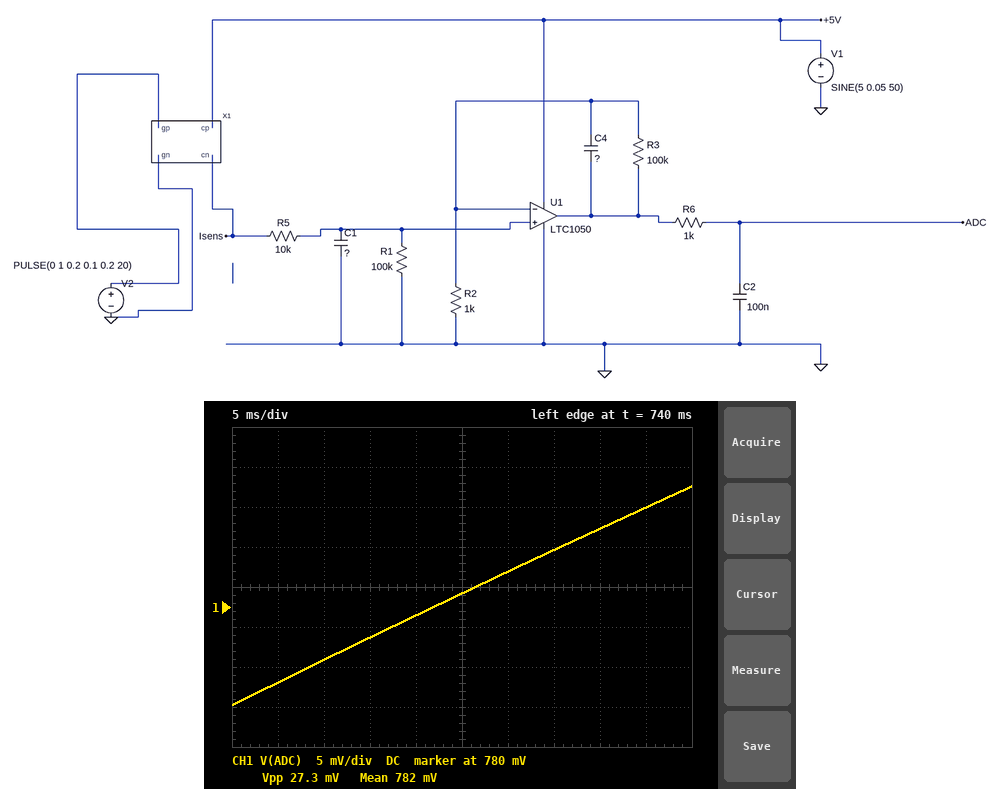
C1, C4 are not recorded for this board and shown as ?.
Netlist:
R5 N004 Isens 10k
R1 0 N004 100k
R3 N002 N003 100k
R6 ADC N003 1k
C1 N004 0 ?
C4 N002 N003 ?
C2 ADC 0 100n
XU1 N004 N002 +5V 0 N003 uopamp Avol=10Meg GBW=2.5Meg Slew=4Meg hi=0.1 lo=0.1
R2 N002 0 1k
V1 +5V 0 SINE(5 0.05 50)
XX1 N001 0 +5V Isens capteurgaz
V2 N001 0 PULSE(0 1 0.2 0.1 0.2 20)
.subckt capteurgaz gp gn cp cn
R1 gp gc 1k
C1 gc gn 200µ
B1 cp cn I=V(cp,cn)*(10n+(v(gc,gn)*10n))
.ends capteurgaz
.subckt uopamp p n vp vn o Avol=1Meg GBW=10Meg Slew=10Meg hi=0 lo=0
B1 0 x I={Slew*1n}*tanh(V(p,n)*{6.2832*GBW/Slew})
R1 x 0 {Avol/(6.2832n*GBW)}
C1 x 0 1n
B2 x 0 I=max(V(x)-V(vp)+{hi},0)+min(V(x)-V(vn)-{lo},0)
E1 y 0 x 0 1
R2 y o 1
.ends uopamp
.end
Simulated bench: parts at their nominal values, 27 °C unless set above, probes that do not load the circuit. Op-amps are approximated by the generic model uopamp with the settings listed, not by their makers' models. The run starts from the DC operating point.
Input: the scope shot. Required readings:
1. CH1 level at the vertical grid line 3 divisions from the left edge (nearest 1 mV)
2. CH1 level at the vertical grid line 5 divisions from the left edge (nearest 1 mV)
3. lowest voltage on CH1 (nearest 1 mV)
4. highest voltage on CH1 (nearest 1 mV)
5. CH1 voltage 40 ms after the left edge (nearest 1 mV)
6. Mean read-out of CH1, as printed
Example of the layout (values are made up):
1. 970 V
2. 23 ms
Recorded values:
1. 776 mV
2. 782 mV
3. 768 mV
4. 795 mV
5. 790 mV
6. 782 mV
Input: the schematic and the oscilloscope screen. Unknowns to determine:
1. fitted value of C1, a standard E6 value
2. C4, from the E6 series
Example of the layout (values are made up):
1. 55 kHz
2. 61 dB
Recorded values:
1. 330 nF
2. 3.3 µF
